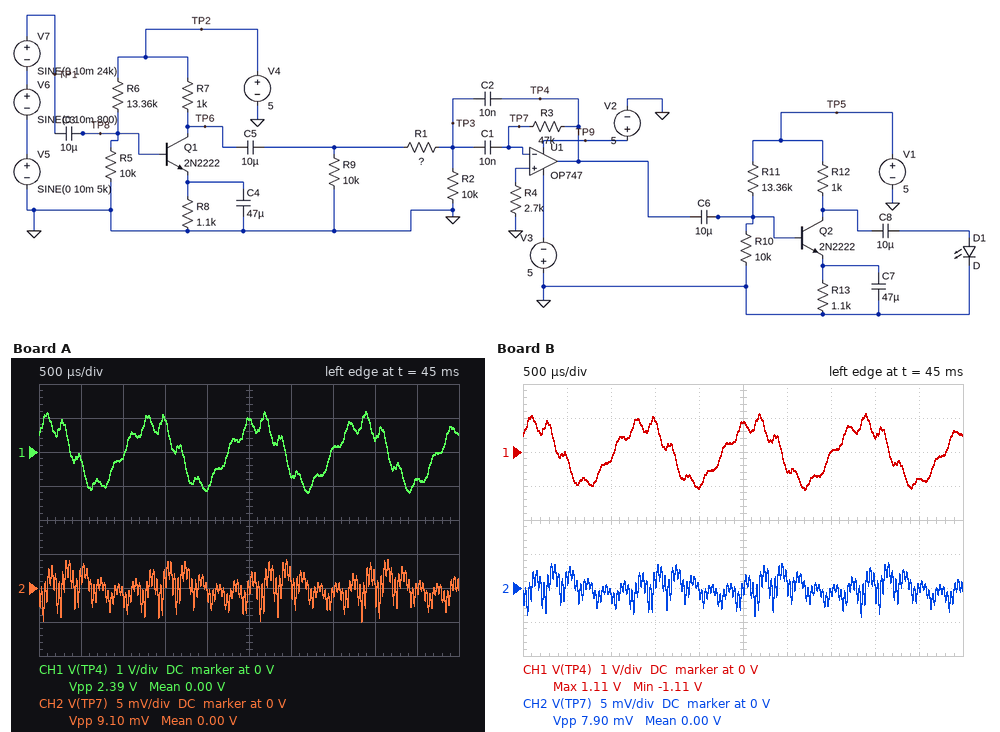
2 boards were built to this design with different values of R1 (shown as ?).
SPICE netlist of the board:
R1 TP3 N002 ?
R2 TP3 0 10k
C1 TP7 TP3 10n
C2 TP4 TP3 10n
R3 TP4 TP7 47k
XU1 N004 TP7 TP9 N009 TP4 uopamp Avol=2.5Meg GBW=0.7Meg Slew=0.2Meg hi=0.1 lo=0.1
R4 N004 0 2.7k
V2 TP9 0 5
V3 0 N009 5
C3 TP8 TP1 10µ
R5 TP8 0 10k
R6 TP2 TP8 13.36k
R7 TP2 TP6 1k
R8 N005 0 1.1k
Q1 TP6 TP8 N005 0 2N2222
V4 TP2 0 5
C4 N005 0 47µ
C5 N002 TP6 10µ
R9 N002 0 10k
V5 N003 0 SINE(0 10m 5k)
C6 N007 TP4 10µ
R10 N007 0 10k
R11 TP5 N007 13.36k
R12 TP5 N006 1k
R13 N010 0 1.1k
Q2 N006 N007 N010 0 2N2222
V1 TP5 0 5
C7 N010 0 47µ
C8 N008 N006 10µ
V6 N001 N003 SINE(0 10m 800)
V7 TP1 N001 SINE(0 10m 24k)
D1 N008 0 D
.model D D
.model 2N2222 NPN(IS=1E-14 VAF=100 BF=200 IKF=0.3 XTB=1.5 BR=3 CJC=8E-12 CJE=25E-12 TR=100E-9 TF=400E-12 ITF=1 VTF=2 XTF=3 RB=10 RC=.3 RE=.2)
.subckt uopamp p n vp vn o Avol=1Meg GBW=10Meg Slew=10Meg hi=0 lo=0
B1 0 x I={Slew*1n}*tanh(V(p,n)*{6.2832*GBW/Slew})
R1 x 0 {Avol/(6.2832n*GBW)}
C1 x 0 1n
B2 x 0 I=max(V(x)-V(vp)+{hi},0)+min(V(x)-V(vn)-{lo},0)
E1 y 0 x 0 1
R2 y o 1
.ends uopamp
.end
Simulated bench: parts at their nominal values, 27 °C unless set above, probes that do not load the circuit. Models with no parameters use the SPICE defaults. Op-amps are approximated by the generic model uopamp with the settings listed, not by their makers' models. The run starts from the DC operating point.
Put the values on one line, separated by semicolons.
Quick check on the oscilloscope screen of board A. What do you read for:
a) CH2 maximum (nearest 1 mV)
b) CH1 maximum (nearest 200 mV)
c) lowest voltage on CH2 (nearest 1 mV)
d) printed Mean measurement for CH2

4 mV; 1.2 V; -5 mV; 0.00 V
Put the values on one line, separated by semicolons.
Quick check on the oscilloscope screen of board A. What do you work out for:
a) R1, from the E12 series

5.6 kΩ
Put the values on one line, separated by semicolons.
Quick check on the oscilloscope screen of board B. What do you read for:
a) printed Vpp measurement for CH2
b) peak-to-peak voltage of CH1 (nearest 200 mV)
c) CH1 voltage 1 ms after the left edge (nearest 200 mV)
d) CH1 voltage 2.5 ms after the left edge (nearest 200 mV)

7.90 mV; 2.2 V; -200 mV; 800 mV
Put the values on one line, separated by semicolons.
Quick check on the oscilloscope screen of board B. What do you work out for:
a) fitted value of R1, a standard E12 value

6.8 kΩ
